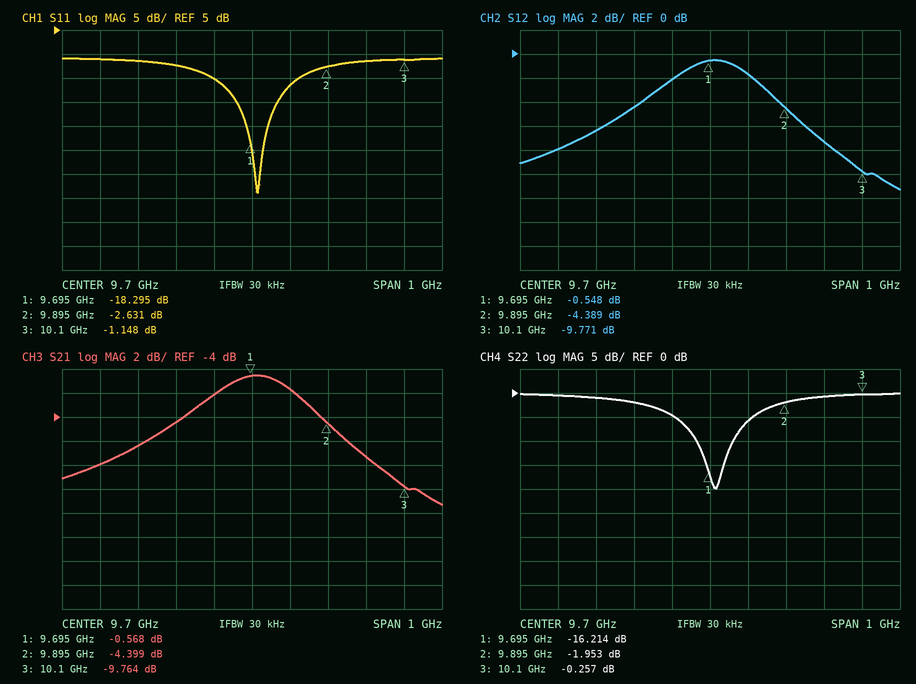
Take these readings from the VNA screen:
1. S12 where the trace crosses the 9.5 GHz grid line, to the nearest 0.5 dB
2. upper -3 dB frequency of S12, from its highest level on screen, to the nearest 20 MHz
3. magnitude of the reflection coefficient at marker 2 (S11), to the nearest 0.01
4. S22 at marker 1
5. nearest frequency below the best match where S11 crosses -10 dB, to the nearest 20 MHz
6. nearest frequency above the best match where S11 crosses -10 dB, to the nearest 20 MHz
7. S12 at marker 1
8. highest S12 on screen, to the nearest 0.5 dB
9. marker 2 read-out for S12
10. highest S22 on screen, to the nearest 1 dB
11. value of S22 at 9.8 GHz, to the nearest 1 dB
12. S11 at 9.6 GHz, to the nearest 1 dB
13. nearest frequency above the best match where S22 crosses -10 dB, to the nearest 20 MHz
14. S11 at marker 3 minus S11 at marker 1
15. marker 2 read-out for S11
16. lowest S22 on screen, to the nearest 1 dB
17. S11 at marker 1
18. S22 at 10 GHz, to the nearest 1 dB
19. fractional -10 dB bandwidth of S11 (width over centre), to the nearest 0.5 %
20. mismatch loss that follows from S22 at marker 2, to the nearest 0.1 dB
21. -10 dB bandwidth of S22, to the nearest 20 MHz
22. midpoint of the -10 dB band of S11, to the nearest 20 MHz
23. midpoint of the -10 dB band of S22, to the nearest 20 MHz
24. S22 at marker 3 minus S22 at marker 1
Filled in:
-4.5 dB
9.86 GHz
0.74
-16.214 dB
9.66 GHz
9.76 GHz
-0.548 dB
-0.5 dB
-4.389 dB
0 dB
-6 dB
-5 dB
9.76 GHz
17.147 dB
-2.631 dB
-20 dB
-18.295 dB
-1 dB
1.0 %
4.4 dB
100 MHz
9.72 GHz
9.72 GHz
15.957 dB
